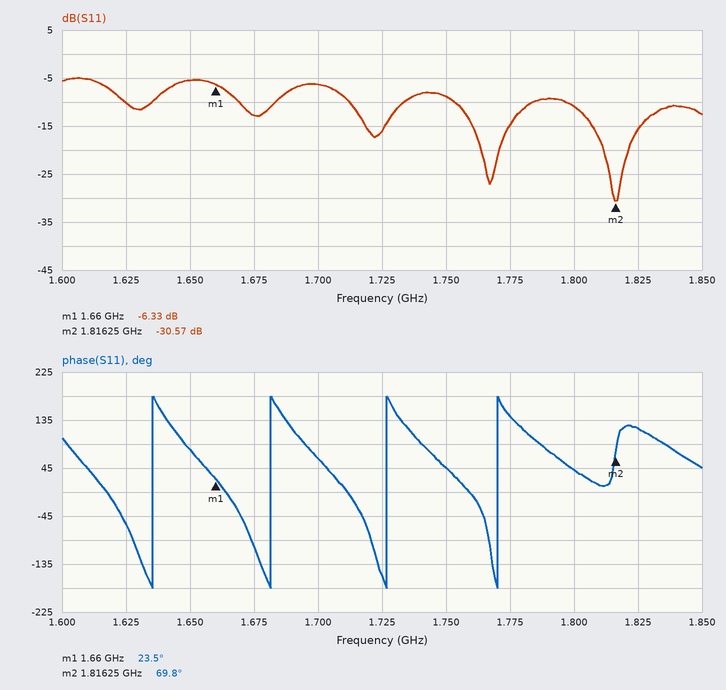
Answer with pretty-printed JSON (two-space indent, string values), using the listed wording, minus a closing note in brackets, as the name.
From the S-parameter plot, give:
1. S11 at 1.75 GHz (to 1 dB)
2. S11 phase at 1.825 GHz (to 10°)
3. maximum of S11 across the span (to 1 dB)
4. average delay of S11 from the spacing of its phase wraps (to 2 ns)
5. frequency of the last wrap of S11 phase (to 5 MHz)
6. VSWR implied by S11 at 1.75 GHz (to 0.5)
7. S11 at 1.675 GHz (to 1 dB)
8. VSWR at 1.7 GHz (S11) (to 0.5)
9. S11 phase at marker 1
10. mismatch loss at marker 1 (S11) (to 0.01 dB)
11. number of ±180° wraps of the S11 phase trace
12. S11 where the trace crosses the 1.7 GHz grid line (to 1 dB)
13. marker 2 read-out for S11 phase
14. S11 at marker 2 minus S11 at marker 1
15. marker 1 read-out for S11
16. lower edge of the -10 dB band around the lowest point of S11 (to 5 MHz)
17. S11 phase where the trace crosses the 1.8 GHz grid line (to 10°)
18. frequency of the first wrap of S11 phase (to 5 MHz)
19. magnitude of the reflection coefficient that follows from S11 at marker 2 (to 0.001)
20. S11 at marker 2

{
  "S11 at 1.75 GHz": "-9 dB",
  "S11 phase at 1.825 GHz": "120°",
  "maximum of S11 across the span": "-5 dB",
  "average delay of S11 from the spacing of its phase wraps": "22 ns",
  "frequency of the last wrap of S11 phase": "1.770 GHz",
  "VSWR implied by S11 at 1.75 GHz": "2.0",
  "S11 at 1.675 GHz": "-13 dB",
  "VSWR at 1.7 GHz (S11)": "3.0",
  "S11 phase at marker 1": "23.5°",
  "mismatch loss at marker 1 (S11)": "1.15 dB",
  "number of ±180° wraps of the S11 phase trace": "4",
  "S11 where the trace crosses the 1.7 GHz grid line": "-6 dB",
  "marker 2 read-out for S11 phase": "69.8°",
  "S11 at marker 2 minus S11 at marker 1": "-24.24 dB",
  "marker 1 read-out for S11": "-6.33 dB",
  "lower edge of the -10 dB band around the lowest point of S11": "1.795 GHz",
  "S11 phase where the trace crosses the 1.8 GHz grid line": "40°",
  "frequency of the first wrap of S11 phase": "1.635 GHz",
  "magnitude of the reflection coefficient that follows from S11 at marker 2": "0.030",
  "S11 at marker 2": "-30.57 dB"
}
